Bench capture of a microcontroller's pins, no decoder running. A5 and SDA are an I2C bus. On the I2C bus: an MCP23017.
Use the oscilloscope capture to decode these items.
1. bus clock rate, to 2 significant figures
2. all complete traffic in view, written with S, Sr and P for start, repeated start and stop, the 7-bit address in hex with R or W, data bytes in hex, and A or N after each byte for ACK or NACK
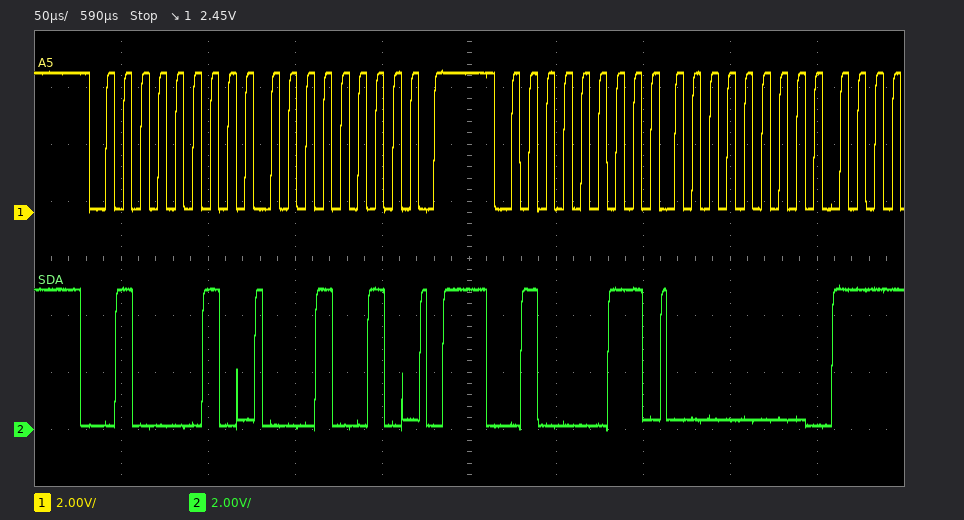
100 kHz
S 21W A 12 A P S 21R A 00 A
